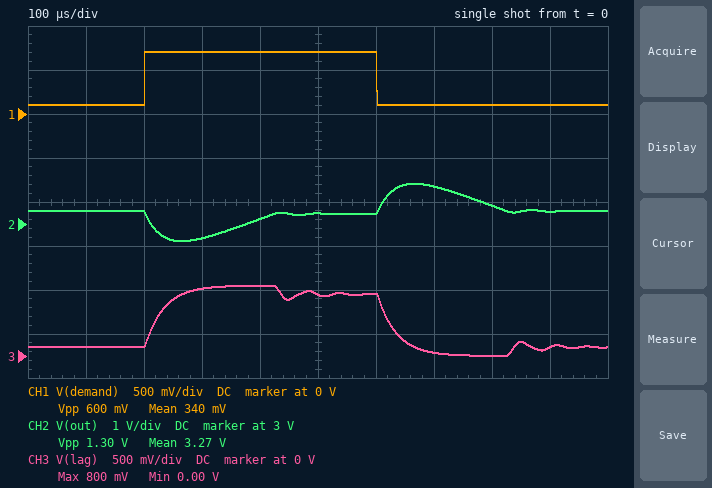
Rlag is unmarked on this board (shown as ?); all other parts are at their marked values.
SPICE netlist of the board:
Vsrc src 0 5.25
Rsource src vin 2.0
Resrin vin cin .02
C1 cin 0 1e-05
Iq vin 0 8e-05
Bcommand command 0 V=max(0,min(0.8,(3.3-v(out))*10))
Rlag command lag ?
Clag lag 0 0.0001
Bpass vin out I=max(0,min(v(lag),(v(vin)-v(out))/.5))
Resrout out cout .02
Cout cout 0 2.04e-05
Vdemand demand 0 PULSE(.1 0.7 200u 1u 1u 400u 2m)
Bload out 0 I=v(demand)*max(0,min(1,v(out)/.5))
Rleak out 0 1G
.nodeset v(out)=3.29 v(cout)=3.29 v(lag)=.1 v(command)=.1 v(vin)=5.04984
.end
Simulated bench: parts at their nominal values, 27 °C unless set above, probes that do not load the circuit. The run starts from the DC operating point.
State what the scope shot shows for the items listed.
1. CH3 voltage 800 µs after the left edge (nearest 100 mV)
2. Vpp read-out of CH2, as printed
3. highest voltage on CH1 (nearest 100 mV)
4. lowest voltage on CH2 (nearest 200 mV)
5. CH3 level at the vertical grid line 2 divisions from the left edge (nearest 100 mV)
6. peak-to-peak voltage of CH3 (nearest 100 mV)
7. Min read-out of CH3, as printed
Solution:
0 V
1.30 V
700 mV
2.6 V
100 mV
800 mV
0.00 V
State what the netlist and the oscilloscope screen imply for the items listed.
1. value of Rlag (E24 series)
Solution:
0.33 Ω
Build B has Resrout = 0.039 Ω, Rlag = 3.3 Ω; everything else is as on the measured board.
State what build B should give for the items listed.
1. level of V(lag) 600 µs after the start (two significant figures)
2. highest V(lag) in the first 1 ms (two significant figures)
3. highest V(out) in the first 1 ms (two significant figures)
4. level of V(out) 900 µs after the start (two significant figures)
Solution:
590 mV
650 mV
5.0 V
4.9 V
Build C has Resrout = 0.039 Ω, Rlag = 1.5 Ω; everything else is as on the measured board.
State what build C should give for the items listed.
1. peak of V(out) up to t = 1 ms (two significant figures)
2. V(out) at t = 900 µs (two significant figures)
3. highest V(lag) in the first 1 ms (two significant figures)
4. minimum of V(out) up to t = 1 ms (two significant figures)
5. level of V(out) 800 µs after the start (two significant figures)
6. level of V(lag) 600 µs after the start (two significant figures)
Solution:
5.0 V
4.9 V
770 mV
460 mV
4.7 V
750 mV
